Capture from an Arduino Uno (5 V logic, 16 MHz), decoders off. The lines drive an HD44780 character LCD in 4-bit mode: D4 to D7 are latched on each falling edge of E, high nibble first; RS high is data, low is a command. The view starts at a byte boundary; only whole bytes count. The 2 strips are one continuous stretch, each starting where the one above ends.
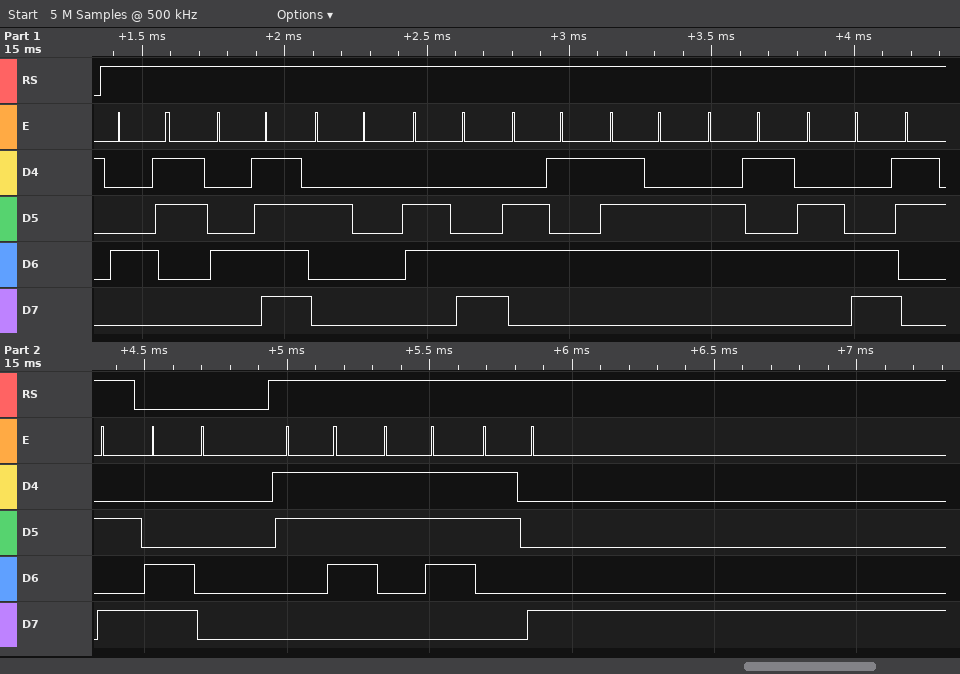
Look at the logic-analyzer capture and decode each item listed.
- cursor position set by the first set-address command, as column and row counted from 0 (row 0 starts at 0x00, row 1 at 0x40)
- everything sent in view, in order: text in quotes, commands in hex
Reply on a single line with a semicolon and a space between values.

column 0, row 1; "CO level:" 0xC0 "778"
